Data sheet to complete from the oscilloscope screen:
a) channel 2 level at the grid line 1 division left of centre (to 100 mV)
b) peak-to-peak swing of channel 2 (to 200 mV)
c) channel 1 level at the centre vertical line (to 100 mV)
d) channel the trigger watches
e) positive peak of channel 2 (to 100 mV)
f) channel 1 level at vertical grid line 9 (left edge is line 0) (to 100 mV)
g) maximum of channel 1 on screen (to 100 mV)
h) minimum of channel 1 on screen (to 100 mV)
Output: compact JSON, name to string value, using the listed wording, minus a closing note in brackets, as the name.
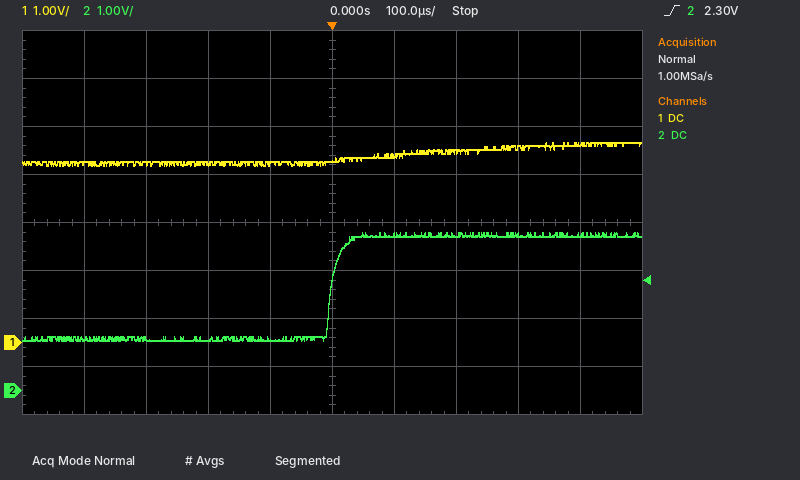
{"channel 2 level at the grid line 1 division left of centre": "1.1 V", "peak-to-peak swing of channel 2": "2.2 V", "channel 1 level at the centre vertical line": "3.8 V", "channel the trigger watches": "channel 2", "positive peak of channel 2": "3.3 V", "channel 1 level at vertical grid line 9 (left edge is line 0)": "4.1 V", "maximum of channel 1 on screen": "4.2 V", "minimum of channel 1 on screen": "3.7 V"}
